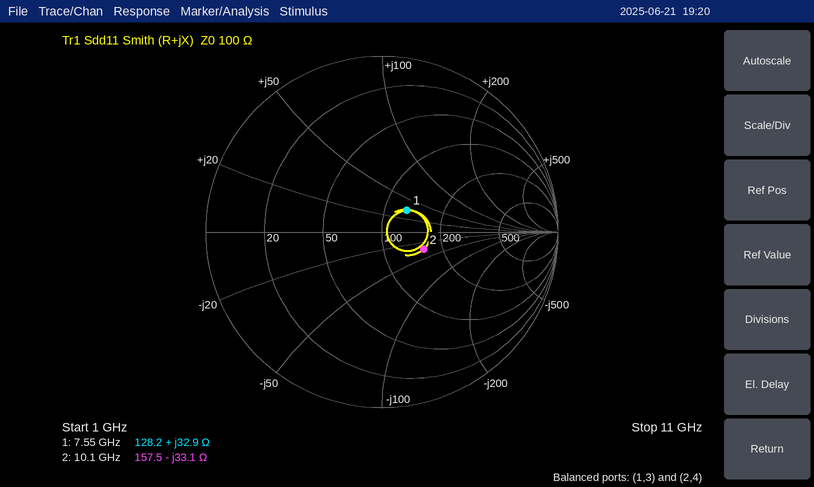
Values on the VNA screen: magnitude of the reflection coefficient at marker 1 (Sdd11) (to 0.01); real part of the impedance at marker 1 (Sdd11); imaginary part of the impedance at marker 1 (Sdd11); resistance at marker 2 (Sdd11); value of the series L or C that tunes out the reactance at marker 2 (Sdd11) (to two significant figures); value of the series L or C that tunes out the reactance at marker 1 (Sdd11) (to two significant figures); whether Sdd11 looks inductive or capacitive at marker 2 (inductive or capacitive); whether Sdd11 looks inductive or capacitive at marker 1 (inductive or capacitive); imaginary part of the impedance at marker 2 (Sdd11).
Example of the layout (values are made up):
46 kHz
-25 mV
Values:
0.19
128.2 Ω
+32.9 Ω
157.5 Ω
520 pH
640 fF
capacitive
inductive
-33.1 Ω
